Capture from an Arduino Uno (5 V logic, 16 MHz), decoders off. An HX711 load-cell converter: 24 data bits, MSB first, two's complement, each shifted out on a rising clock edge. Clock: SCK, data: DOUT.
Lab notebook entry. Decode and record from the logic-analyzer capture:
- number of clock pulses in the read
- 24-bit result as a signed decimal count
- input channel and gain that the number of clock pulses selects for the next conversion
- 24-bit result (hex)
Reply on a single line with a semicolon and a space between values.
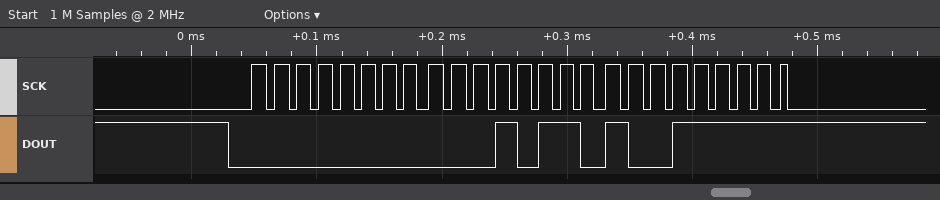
25; 5791; channel A, gain 128; 0x00169F
